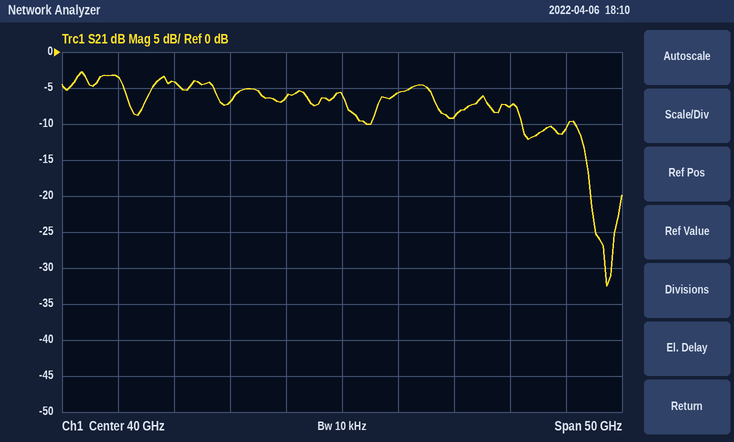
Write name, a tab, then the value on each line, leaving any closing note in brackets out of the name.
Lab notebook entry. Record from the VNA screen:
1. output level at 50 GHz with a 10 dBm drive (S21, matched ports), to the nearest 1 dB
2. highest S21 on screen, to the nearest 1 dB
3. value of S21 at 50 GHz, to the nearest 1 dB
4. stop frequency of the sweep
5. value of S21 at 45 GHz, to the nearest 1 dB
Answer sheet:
output level at 50 GHz with a 10 dBm drive (S21, matched ports), to the nearest 1 dB	1 dBm
highest S21 on screen, to the nearest 1 dB	-3 dB
value of S21 at 50 GHz, to the nearest 1 dB	-9 dB
stop frequency of the sweep	65 GHz
value of S21 at 45 GHz, to the nearest 1 dB	-6 dB
